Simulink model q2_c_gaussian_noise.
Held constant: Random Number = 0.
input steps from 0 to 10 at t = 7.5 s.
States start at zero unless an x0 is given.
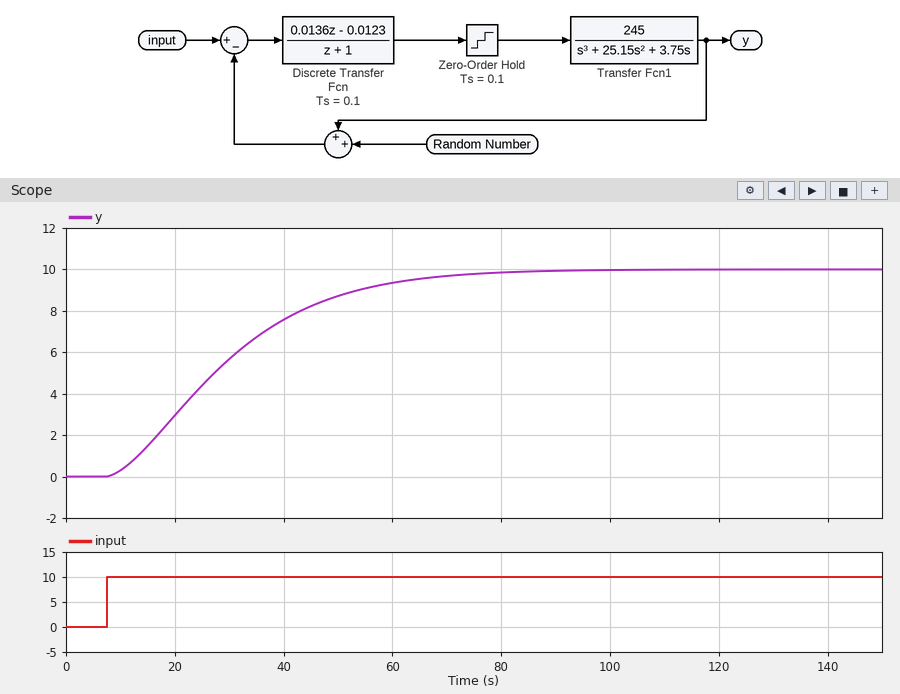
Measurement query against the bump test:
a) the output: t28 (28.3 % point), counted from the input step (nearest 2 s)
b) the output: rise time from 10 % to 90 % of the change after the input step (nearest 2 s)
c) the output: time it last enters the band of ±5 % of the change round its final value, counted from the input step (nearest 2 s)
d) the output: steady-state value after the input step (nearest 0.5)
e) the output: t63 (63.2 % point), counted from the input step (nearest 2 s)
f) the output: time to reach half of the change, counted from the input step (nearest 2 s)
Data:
12 s
40 s
56 s
10.0
26 s
20 s
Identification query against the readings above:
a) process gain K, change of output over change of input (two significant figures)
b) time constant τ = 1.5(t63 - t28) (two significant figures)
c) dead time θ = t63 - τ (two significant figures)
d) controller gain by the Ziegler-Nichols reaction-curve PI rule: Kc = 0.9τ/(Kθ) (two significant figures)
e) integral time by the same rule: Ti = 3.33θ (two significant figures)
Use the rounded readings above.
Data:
1.0
21 s
5.0 s
3.8
17 s
